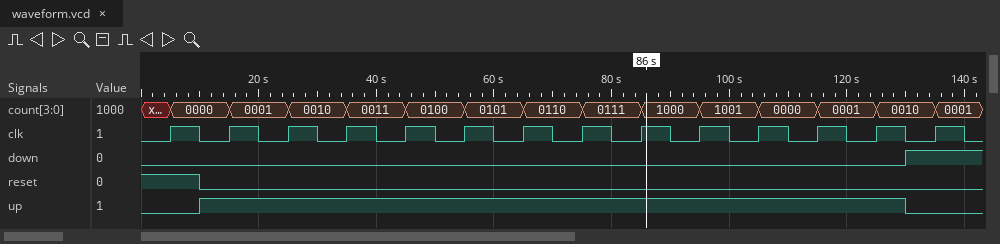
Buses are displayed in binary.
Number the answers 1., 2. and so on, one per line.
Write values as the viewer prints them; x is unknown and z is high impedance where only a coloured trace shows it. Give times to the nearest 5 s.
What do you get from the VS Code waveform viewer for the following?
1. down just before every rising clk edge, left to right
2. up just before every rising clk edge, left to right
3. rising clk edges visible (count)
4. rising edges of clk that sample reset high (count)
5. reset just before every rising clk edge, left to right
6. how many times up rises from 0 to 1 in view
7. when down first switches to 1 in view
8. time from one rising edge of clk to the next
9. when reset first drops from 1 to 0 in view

1. 0 0 0 0 0 0 0 0 0 0 0 0 0 1
2. 0 1 1 1 1 1 1 1 1 1 1 1 1 0
3. 14
4. 1
5. 1 0 0 0 0 0 0 0 0 0 0 0 0 0
6. 1
7. 130 s
8. 10 s
9. 10 s
